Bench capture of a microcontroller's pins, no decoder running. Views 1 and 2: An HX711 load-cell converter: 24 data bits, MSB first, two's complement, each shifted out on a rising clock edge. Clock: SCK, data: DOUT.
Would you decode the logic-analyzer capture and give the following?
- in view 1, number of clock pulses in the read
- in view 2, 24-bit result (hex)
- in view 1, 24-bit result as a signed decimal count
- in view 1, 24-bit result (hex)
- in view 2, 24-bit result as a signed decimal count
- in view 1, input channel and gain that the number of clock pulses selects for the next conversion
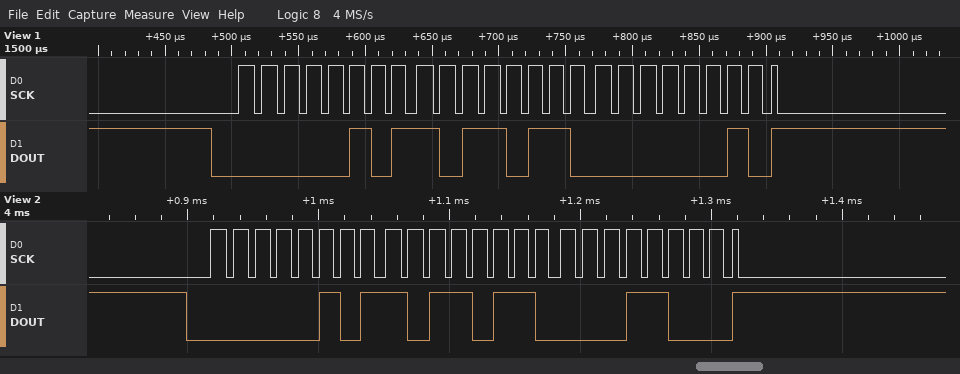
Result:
25
0x05B618
374274
0x05B602
374296
channel A, gain 128
